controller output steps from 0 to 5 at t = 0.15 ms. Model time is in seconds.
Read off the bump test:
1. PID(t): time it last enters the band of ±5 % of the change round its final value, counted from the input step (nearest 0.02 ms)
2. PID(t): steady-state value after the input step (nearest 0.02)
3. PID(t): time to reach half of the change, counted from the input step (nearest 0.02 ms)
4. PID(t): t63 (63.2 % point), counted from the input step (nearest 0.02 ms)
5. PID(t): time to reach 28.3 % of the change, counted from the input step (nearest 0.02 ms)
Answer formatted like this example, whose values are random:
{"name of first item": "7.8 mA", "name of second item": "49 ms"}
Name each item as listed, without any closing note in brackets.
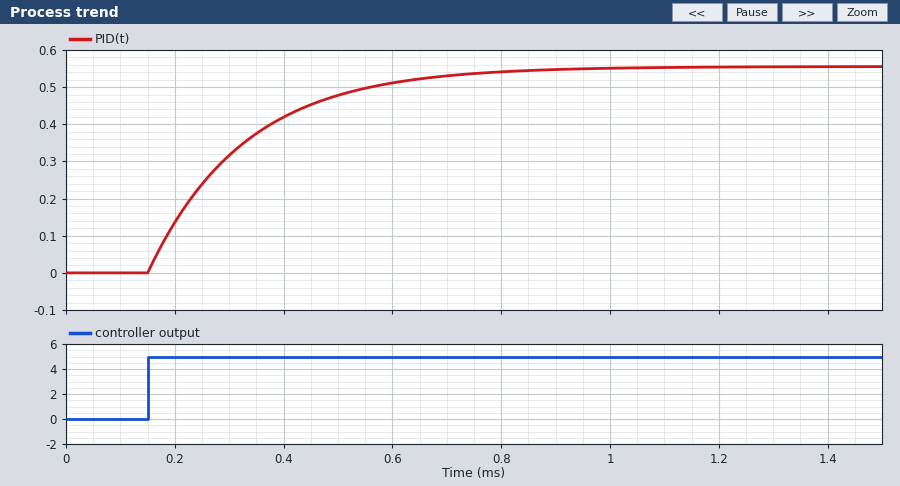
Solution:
{"PID(t): time it last enters the band of ±5 % of the change round its final value, counted from the input step": "0.54 ms", "PID(t): steady-state value after the input step": "0.56", "PID(t): time to reach half of the change, counted from the input step": "0.12 ms", "PID(t): t63 (63.2 % point), counted from the input step": "0.18 ms", "PID(t): time to reach 28.3 % of the change, counted from the input step": "0.06 ms"}
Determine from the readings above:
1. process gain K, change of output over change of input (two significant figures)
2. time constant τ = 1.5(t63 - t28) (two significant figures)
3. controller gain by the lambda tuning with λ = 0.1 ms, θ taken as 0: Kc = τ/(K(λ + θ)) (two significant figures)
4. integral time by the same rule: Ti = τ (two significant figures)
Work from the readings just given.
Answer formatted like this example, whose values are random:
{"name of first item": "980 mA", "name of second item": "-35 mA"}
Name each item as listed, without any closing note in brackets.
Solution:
{"process gain K, change of output over change of input": "0.11", "time constant τ = 1.5(t63 - t28)": "0.18 ms", "controller gain by the lambda tuning with λ = 0.1 ms, θ taken as 0: Kc = τ/(K(λ + θ))": "16", "integral time by the same rule: Ti = τ": "0.18 ms"}
